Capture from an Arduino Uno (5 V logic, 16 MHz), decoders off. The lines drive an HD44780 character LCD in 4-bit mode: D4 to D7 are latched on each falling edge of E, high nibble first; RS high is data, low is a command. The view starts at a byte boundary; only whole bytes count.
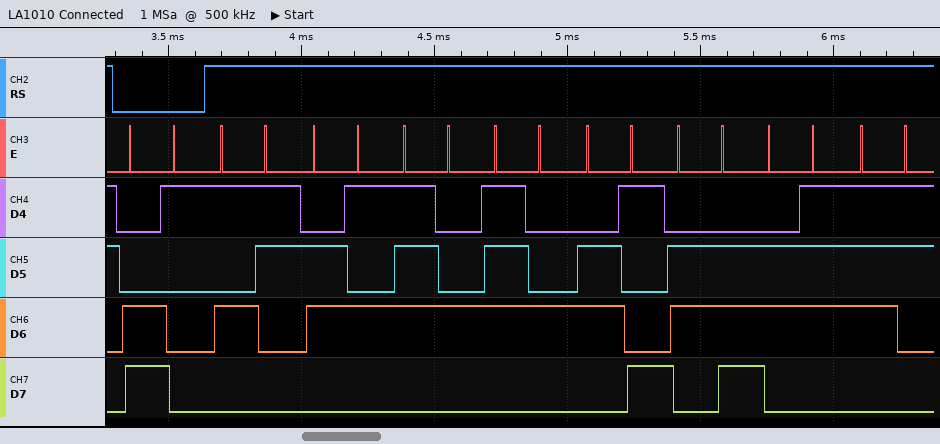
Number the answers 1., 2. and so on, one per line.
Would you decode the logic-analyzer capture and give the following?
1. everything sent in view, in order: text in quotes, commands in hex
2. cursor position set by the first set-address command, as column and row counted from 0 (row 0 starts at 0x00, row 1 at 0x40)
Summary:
1. 0xC1 "Settings"
2. column 1, row 1
